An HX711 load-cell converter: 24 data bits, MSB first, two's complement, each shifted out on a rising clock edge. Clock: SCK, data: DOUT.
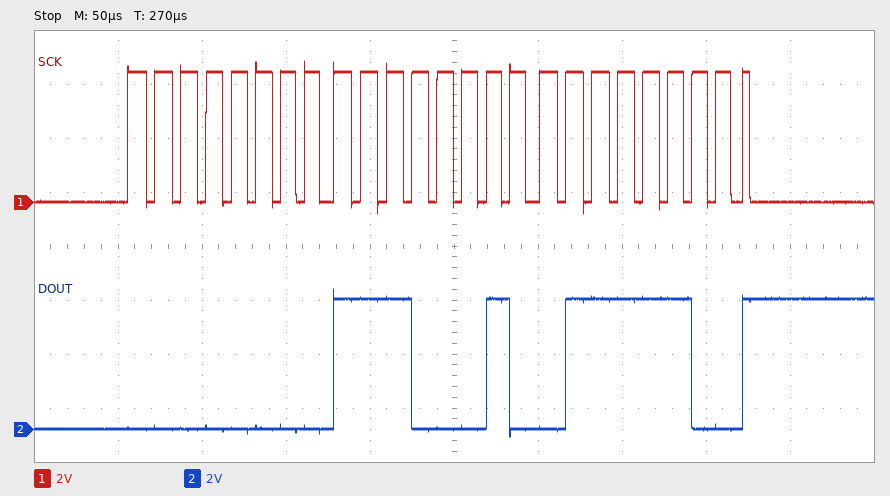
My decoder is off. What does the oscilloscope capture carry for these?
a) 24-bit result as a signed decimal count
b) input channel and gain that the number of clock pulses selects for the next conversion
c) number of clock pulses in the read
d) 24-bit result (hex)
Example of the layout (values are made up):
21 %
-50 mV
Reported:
57980
channel A, gain 128
25
0x00E27C
